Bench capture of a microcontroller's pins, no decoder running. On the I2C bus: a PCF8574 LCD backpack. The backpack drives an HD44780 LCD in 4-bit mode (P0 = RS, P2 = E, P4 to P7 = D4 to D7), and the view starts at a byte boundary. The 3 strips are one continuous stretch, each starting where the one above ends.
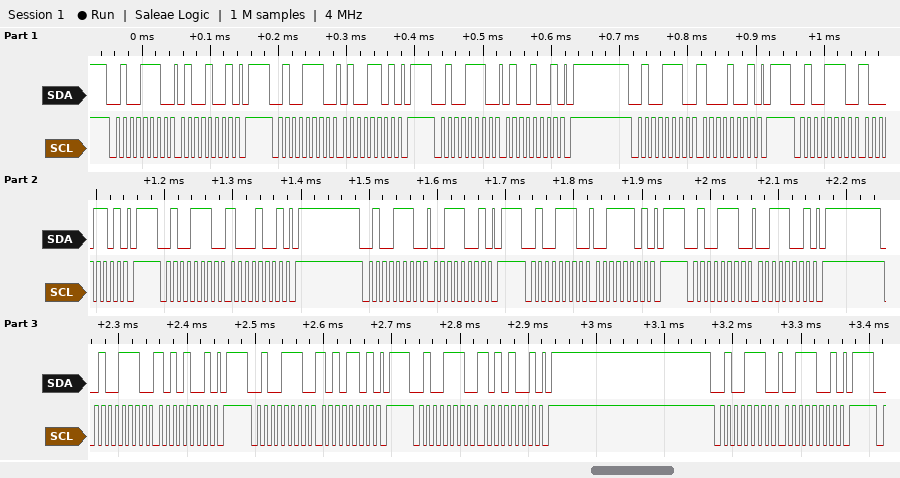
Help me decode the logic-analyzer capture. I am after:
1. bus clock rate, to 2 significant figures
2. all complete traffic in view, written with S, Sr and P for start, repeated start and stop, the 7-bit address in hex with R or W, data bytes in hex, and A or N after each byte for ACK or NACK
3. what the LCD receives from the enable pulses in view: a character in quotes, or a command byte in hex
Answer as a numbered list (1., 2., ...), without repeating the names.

1. 100 kHz
2. S 27W A 49 A P S 27W A 4D A P S 27W A 49 A P S 27W A 89 A P S 27W A 8D A P S 27W A 89 A P S 27W A 39 A P S 27W A 3D A P S 27W A 39 A P S 27W A A9 A P S 27W A AD A P S 27W A A9 A P S 27W A 39 A P
3. 'H' ':'
